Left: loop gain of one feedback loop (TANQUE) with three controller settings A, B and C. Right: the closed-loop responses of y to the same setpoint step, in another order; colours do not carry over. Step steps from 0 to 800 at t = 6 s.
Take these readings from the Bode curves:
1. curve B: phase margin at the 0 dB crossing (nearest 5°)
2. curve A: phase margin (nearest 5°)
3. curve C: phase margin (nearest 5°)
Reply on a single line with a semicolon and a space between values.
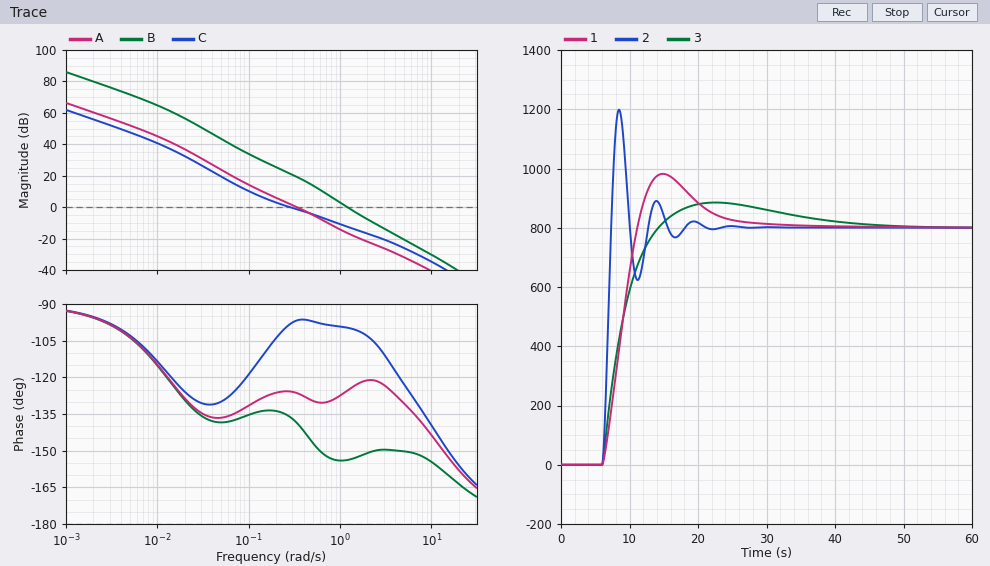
25°; 55°; 80°
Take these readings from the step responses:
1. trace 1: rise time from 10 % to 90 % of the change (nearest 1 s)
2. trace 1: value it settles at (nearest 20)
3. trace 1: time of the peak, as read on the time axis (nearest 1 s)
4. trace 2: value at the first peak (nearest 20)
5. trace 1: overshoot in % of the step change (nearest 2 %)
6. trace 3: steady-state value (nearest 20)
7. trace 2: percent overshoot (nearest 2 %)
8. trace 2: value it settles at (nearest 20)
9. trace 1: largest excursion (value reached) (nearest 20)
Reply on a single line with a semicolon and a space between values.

4 s; 800; 15 s; 1200; 22 %; 800; 50 %; 800; 980
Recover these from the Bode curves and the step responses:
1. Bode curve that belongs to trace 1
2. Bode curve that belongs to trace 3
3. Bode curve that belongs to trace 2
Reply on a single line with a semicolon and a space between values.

A; C; B
